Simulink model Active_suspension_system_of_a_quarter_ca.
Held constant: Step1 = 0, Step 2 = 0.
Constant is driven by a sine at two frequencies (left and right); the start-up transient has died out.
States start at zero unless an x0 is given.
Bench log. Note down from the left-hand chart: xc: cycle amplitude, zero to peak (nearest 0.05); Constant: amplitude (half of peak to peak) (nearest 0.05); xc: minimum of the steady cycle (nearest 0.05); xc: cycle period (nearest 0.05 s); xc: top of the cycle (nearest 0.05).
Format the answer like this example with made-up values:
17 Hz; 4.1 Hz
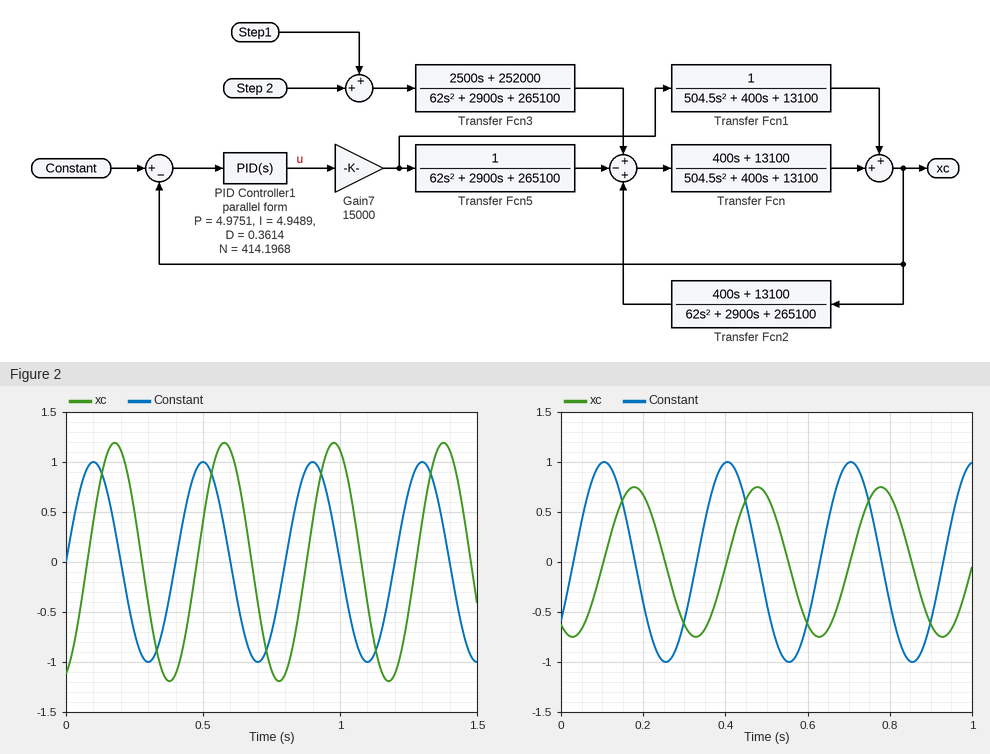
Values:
1.20; 1.00; -1.20; 0.40 s; 1.20
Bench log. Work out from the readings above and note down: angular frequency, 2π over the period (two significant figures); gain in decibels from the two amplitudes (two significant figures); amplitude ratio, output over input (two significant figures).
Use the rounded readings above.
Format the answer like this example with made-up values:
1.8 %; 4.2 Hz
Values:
16 rad/s; 1.6 dB; 1.2
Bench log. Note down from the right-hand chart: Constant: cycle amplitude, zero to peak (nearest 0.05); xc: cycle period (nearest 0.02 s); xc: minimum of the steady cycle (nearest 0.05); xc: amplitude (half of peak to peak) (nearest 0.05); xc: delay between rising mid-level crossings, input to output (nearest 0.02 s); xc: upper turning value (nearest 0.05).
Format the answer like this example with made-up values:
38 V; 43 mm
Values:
1.00; 0.30 s; -0.75; 0.75; 0.08 s; 0.75
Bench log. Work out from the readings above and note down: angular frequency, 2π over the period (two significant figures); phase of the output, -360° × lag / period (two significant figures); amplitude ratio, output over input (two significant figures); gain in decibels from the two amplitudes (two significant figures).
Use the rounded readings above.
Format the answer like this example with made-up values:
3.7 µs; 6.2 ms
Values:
21 rad/s; -96°; 0.75; -2.5 dB
